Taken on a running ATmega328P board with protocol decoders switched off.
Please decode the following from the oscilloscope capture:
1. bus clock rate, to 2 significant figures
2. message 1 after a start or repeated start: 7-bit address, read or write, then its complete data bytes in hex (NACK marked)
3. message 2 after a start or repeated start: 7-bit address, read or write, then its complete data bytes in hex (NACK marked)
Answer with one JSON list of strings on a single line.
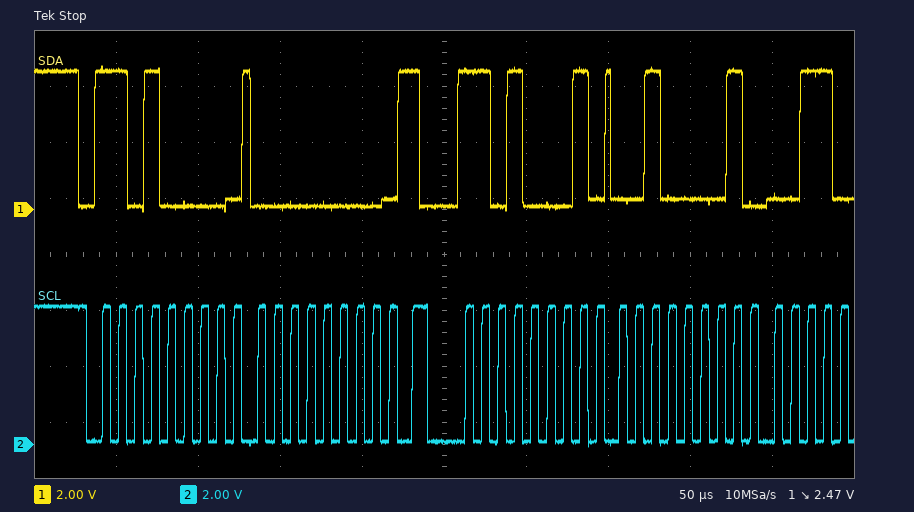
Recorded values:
["100 kHz", "0x68 write: 00", "0x68 read: 21"]
